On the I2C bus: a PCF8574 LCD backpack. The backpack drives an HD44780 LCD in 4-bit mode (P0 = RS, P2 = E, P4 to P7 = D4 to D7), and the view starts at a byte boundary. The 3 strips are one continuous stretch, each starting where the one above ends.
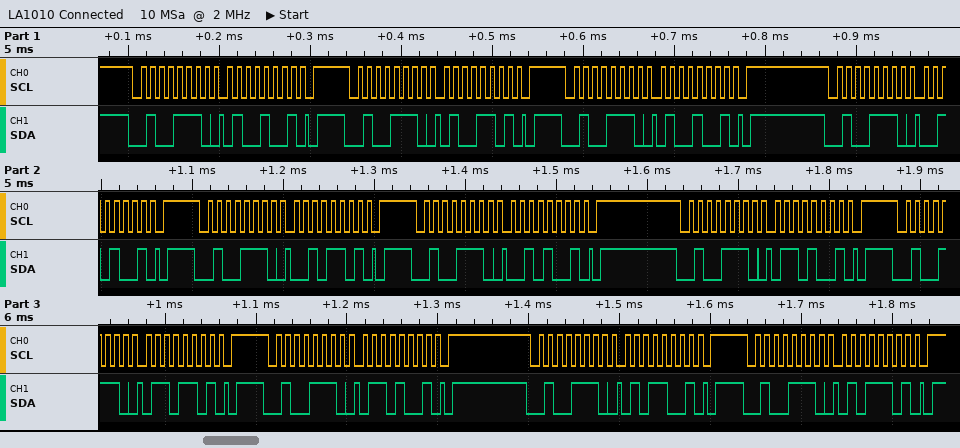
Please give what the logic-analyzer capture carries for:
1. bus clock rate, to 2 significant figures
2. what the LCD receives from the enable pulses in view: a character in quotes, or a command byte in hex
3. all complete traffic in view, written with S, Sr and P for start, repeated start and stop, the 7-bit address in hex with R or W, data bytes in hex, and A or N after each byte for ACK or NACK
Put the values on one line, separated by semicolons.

100 kHz; 'B'; S 27W A 49 A P S 27W A 4D A P S 27W A 49 A P S 27W A 29 A P S 27W A 2D A P S 27W A 29 A P S 27W A 69 A P S 27W A 6D A P S 27W A 69 A P S 27W A 59 A P S 27W A 5D A P
